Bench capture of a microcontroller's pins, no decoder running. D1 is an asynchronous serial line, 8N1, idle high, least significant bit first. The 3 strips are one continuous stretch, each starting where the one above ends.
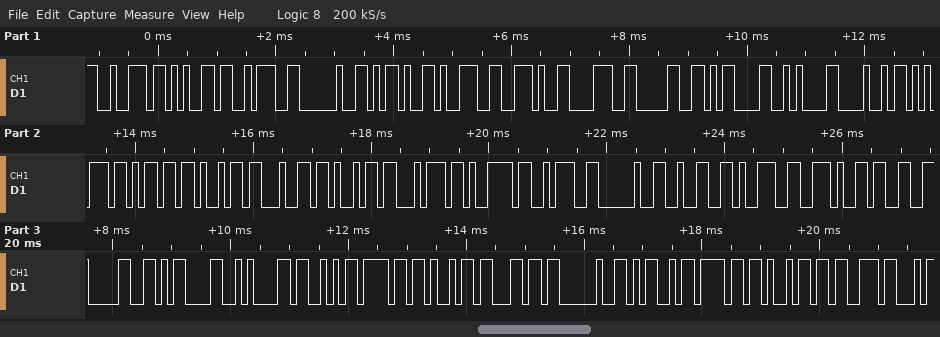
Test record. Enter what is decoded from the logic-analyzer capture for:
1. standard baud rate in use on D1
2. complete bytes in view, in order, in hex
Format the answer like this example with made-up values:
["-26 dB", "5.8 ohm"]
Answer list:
["9600 baud", "72 65 3A 20 2D 39 2E 38 30 0D 0A 48 75 6D 69 64 69 74 79 3A 20 32 39 2E 33 30 0D 0A 53 6F 69 6C 20 4D 6F 69 73"]
